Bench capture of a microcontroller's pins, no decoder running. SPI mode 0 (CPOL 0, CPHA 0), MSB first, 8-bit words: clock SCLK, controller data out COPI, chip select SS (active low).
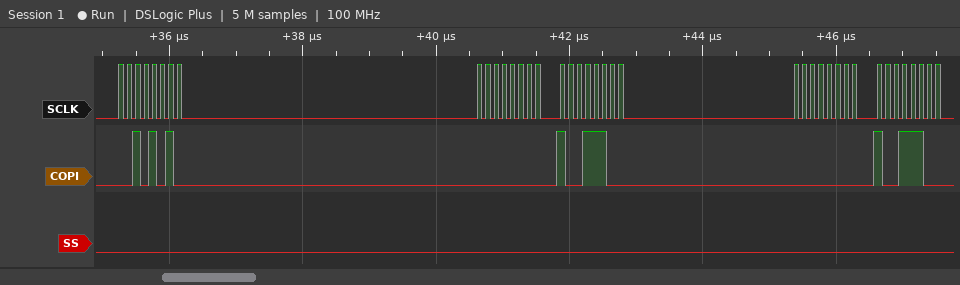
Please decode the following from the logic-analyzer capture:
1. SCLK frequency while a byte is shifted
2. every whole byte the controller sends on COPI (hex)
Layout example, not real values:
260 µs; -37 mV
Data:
8 MHz; 0x2A 0x00 0x9C 0x00 0x9C
